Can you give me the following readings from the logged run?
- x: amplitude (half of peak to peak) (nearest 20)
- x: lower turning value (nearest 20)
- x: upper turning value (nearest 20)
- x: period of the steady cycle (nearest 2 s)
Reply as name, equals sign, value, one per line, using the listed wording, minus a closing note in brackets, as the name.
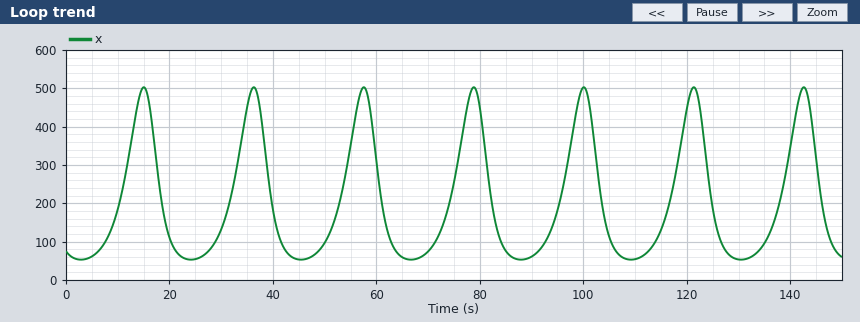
x: amplitude (half of peak to peak) = 220
x: lower turning value = 60
x: upper turning value = 500
x: period of the steady cycle = 22 s
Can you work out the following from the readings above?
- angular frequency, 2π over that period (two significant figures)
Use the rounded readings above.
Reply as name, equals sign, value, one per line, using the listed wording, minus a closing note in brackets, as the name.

angular frequency, 2π over that period = 0.29 rad/s
